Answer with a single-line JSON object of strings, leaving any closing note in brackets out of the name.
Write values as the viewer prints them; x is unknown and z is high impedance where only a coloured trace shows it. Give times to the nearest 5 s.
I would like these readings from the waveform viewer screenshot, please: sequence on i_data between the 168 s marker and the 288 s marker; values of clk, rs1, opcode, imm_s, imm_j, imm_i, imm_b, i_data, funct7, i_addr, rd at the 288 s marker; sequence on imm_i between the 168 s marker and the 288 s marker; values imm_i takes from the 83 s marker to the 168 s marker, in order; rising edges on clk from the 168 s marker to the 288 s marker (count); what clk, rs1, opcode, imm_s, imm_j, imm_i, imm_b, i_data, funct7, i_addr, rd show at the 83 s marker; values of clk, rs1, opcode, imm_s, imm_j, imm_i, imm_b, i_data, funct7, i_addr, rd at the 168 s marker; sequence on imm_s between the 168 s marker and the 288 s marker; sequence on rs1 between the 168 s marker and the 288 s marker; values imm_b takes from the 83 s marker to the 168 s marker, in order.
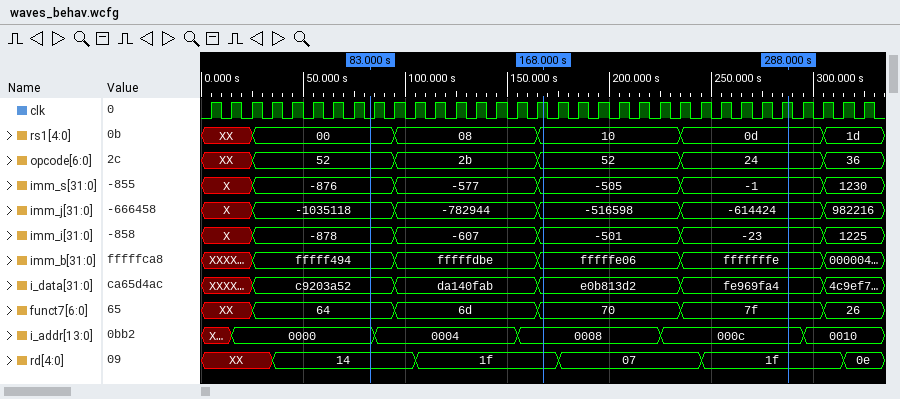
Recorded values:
{"sequence on i_data between the 168 s marker and the 288 s marker": "e0b813d2, fe969fa4", "values of clk, rs1, opcode, imm_s, imm_j, imm_i, imm_b, i_data, funct7, i_addr, rd at the 288 s marker": "clk=1, rs1=0d, opcode=24, imm_s=-1, imm_j=-614424, imm_i=-23, imm_b=fffffffe, i_data=fe969fa4, funct7=7f, i_addr=000c, rd=1f", "sequence on imm_i between the 168 s marker and the 288 s marker": "-501, -23", "values imm_i takes from the 83 s marker to the 168 s marker, in order": "-878, -607, -501", "rising edges on clk from the 168 s marker to the 288 s marker": "12", "what clk, rs1, opcode, imm_s, imm_j, imm_i, imm_b, i_data, funct7, i_addr, rd show at the 83 s marker": "clk=0, rs1=00, opcode=52, imm_s=-876, imm_j=-1035118, imm_i=-878, imm_b=fffff494, i_data=c9203a52, funct7=64, i_addr=0000, rd=14", "values of clk, rs1, opcode, imm_s, imm_j, imm_i, imm_b, i_data, funct7, i_addr, rd at the 168 s marker": "clk=1, rs1=10, opcode=52, imm_s=-505, imm_j=-516598, imm_i=-501, imm_b=fffffe06, i_data=e0b813d2, funct7=70, i_addr=0008, rd=1f", "sequence on imm_s between the 168 s marker and the 288 s marker": "-505, -1", "sequence on rs1 between the 168 s marker and the 288 s marker": "10, 0d", "values imm_b takes from the 83 s marker to the 168 s marker, in order": "fffff494, fffffdbe, fffffe06"}
